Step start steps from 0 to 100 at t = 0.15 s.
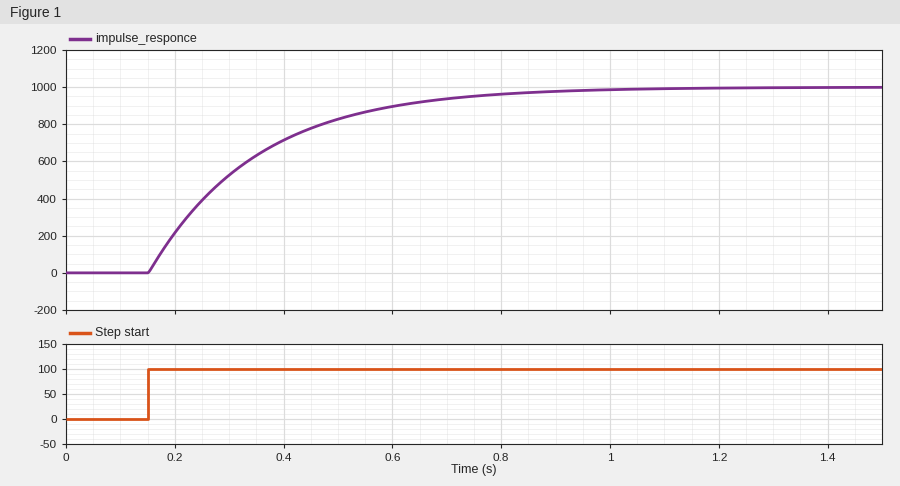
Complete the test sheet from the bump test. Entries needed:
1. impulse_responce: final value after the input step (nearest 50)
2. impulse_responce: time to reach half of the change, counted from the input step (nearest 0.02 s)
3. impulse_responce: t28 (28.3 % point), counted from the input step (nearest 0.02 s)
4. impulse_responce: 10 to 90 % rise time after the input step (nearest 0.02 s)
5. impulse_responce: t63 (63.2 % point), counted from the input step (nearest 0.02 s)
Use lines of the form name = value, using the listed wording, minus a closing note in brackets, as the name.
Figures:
impulse_responce: final value after the input step = 1000
impulse_responce: time to reach half of the change, counted from the input step = 0.14 s
impulse_responce: t28 (28.3 % point), counted from the input step = 0.06 s
impulse_responce: 10 to 90 % rise time after the input step = 0.44 s
impulse_responce: t63 (63.2 % point), counted from the input step = 0.20 s
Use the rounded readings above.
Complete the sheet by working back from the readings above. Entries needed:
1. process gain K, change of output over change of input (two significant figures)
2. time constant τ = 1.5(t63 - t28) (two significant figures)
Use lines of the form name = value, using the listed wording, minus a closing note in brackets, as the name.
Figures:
process gain K, change of output over change of input = 10
time constant τ = 1.5(t63 - t28) = 0.21 s
